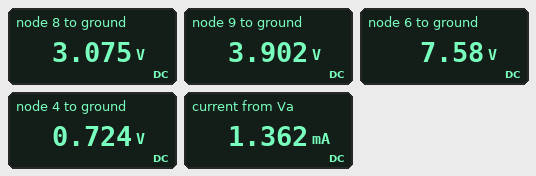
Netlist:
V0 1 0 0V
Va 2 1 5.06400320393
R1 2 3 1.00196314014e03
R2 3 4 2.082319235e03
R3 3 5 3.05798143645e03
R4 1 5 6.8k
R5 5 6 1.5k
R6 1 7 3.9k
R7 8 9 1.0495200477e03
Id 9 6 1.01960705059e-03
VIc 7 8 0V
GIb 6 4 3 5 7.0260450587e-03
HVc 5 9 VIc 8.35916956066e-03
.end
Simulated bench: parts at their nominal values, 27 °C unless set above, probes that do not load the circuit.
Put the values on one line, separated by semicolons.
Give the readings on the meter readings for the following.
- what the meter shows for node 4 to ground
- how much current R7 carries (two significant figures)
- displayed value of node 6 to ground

0.724 V; 790 µA; 7.58 V
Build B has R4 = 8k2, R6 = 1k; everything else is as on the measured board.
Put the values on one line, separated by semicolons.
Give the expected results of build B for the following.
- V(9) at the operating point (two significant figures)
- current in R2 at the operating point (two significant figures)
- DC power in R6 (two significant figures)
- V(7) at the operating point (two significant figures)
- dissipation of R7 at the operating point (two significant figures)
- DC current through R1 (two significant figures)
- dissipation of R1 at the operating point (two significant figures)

3.3 V; 2.1 mA; 2.6 mW; 1.6 V; 2.8 mW; 2.0 mA; 4.1 mW
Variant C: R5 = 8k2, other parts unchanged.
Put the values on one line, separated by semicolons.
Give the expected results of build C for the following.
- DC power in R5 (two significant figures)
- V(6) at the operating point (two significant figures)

49 mW; 24 V
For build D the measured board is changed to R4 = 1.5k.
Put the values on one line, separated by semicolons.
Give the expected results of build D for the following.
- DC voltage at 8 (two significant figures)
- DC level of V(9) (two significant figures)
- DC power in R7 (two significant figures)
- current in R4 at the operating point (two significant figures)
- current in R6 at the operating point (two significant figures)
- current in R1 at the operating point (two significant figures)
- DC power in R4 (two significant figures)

2.3 V; 2.9 V; 360 µW; 1.9 mA; 590 µA; 2.5 mA; 5.6 mW
